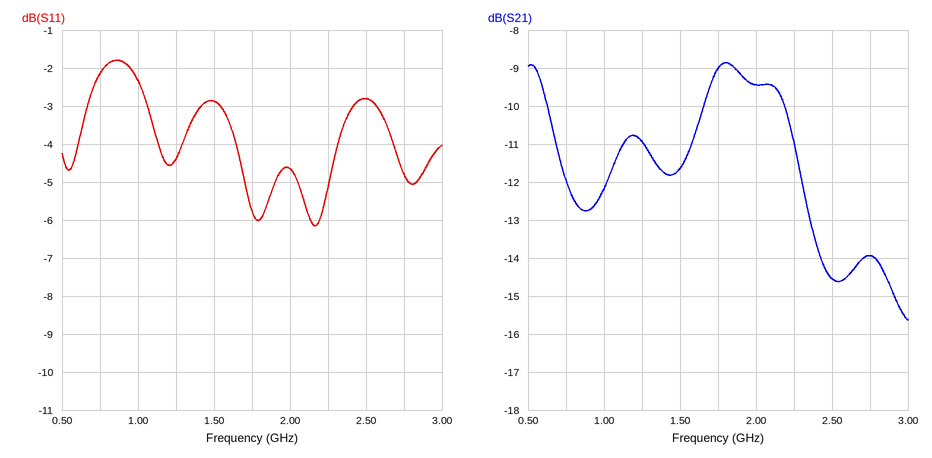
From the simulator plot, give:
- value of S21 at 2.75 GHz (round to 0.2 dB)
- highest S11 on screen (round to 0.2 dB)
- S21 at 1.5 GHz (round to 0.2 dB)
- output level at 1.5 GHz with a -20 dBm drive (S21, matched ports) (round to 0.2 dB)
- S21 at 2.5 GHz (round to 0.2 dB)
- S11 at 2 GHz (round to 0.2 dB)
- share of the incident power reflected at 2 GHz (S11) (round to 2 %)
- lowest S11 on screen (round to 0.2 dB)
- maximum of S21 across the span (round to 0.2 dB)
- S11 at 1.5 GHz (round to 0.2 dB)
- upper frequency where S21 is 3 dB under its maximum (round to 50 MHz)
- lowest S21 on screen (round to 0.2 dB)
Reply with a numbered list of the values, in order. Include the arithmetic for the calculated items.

1. -14.0 dB
2. -1.8 dB
3. -11.6 dB
4. -20 dBm + (-11.6 dB) = -31.6 dBm
5. -14.6 dB
6. -4.6 dB
7. 10^(-4.6/10) ≈ 34.7 %, so 34 % to the nearest 2 %
8. -6.2 dB
9. -8.8 dB
10. -2.8 dB
11. 2.30 GHz
12. -15.6 dB
